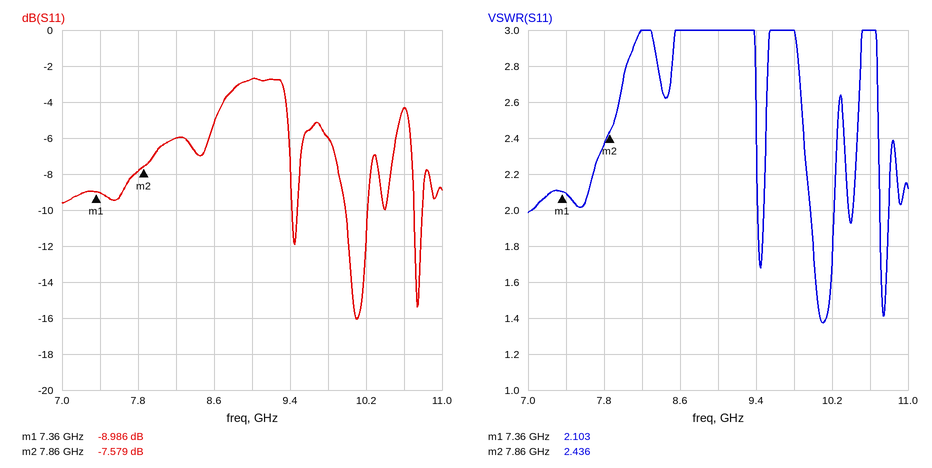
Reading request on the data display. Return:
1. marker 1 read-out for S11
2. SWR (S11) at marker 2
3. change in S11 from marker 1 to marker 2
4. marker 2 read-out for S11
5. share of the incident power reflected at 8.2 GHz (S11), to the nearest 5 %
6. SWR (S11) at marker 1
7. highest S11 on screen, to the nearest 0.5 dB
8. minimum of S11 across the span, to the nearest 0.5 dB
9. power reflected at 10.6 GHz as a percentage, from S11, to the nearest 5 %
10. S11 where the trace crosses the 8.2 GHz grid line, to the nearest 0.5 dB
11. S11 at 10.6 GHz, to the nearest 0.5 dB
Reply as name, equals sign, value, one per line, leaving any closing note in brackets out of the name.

marker 1 read-out for S11 = -8.986 dB
SWR (S11) at marker 2 = 2.436
change in S11 from marker 1 to marker 2 = 1.407 dB
marker 2 read-out for S11 = -7.579 dB
share of the incident power reflected at 8.2 GHz (S11), to the nearest 5 % = 25 %
SWR (S11) at marker 1 = 2.103
highest S11 on screen, to the nearest 0.5 dB = -2.5 dB
minimum of S11 across the span, to the nearest 0.5 dB = -16.0 dB
power reflected at 10.6 GHz as a percentage, from S11, to the nearest 5 % = 35 %
S11 where the trace crosses the 8.2 GHz grid line, to the nearest 0.5 dB = -6.0 dB
S11 at 10.6 GHz, to the nearest 0.5 dB = -4.5 dB
